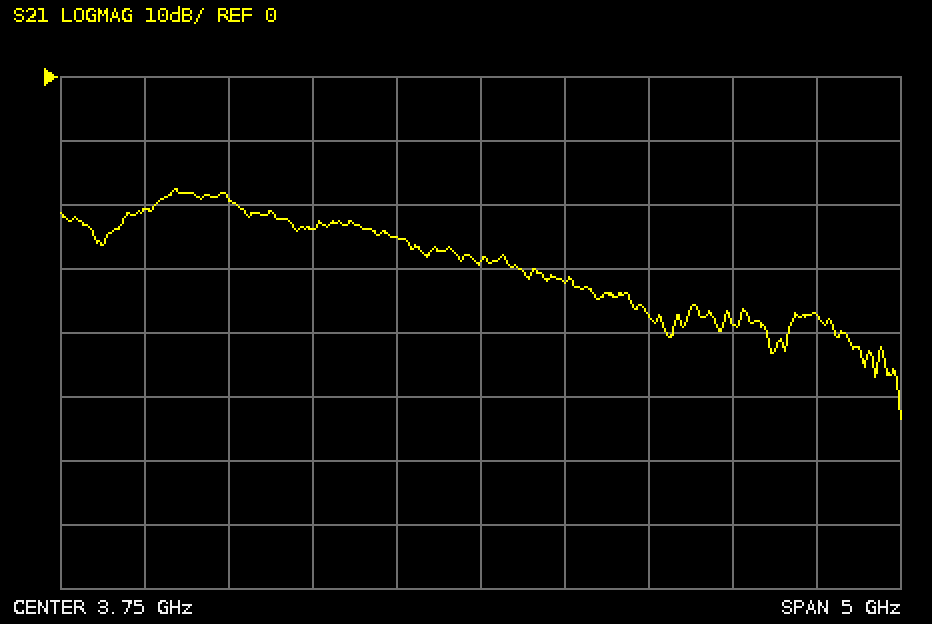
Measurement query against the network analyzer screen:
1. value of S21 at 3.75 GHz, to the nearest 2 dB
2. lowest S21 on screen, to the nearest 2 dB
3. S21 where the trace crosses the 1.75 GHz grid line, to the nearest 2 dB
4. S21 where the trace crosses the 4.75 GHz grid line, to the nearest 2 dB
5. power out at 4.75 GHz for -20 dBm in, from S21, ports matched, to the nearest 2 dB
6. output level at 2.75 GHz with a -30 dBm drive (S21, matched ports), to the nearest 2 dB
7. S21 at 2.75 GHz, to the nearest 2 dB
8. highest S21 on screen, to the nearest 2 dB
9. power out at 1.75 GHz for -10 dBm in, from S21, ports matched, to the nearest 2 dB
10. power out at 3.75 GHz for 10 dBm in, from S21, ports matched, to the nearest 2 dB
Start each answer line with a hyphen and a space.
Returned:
- -28 dB
- -54 dB
- -20 dB
- -38 dB
- -58 dBm
- -54 dBm
- -24 dB
- -18 dB
- -30 dBm
- -18 dBm
